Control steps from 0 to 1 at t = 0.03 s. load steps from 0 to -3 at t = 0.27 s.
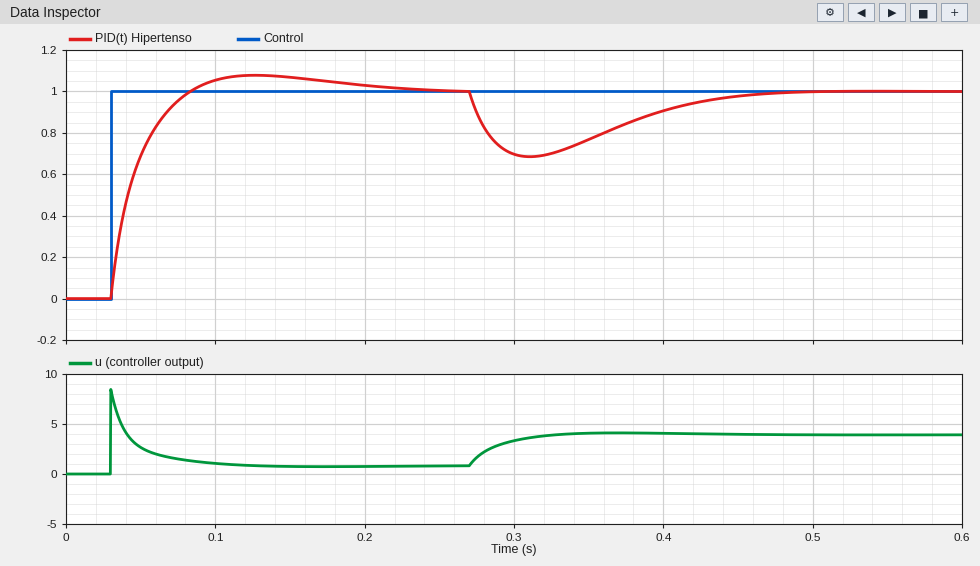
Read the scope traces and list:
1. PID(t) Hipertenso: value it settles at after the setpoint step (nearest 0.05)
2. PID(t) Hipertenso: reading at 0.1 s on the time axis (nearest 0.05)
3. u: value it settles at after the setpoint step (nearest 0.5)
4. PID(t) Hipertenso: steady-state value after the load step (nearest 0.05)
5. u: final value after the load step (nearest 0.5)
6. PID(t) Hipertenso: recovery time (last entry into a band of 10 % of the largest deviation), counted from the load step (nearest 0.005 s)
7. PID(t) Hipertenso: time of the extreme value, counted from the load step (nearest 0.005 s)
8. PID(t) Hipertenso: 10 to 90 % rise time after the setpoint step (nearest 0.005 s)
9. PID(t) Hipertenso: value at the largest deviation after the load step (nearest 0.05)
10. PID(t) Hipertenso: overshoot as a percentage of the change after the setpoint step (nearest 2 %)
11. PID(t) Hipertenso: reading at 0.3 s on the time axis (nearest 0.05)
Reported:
1.00
1.05
1.0
1.00
4.0
0.170 s
0.040 s
0.035 s
0.70
8 %
0.70
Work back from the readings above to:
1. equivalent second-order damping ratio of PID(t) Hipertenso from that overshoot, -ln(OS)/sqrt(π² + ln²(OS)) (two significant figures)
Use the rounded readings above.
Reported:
0.63
